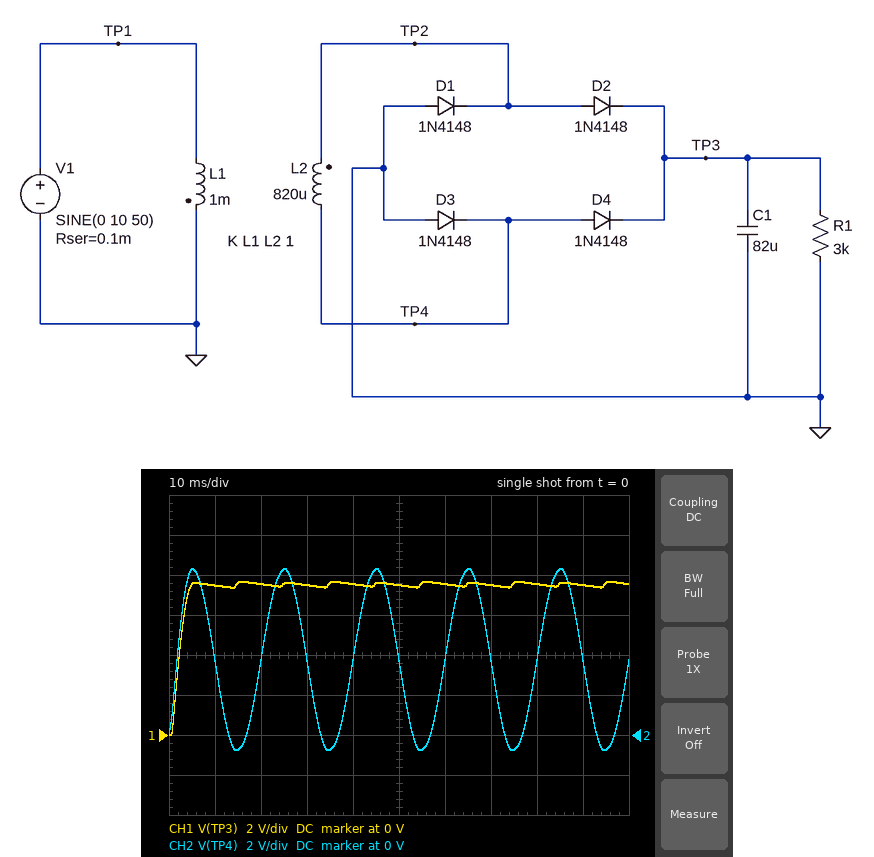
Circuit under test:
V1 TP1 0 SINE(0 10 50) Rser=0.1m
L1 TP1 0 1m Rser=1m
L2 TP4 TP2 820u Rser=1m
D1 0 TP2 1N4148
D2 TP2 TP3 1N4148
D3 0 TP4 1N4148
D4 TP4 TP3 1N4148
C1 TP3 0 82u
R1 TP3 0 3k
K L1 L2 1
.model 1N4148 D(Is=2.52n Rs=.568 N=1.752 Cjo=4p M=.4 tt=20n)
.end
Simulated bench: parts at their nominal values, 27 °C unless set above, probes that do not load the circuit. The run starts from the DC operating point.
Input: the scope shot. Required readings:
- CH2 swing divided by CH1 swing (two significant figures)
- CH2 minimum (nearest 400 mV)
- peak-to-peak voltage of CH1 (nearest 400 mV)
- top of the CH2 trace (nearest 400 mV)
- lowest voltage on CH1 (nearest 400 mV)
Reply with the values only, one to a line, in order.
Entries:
1.2
-800 mV
7.6 V
8.4 V
0 V
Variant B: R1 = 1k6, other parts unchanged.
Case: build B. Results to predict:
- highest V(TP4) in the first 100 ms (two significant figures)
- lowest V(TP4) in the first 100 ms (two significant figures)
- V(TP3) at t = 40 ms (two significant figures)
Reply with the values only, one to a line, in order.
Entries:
8.3 V
-790 mV
7.4 V
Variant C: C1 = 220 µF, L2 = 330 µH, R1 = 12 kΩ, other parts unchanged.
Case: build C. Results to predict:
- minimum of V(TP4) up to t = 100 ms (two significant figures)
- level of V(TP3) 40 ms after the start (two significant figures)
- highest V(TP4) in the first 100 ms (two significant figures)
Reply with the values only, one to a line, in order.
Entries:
-740 mV
4.4 V
5.1 V
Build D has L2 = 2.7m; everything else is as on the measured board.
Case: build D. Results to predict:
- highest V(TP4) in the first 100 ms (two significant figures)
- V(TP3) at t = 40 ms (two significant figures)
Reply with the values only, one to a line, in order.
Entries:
16 V
15 V
